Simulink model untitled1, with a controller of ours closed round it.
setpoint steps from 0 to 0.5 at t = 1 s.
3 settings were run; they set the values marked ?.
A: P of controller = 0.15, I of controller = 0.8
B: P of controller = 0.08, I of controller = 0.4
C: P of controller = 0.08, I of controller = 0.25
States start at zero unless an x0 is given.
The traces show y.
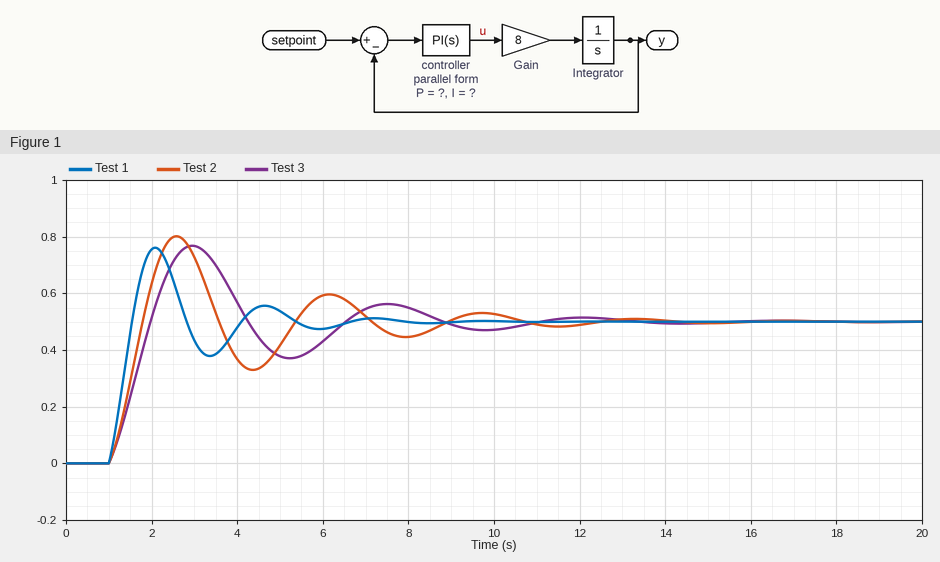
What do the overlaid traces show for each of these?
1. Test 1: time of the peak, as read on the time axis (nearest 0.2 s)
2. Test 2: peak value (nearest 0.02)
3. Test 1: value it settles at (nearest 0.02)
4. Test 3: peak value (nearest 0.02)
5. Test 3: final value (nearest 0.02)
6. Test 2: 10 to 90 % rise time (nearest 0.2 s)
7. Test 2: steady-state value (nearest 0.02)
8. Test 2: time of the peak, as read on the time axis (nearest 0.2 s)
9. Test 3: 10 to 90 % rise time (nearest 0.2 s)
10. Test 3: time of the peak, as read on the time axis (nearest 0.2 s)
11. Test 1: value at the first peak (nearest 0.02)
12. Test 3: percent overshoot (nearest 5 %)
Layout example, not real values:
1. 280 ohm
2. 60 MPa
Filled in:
1. 2.0 s
2. 0.80
3. 0.50
4. 0.76
5. 0.50
6. 0.6 s
7. 0.50
8. 2.6 s
9. 0.8 s
10. 3.0 s
11. 0.76
12. 55 %
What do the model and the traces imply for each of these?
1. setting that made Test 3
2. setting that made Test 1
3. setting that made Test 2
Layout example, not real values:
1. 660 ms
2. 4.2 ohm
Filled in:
1. C
2. A
3. B
